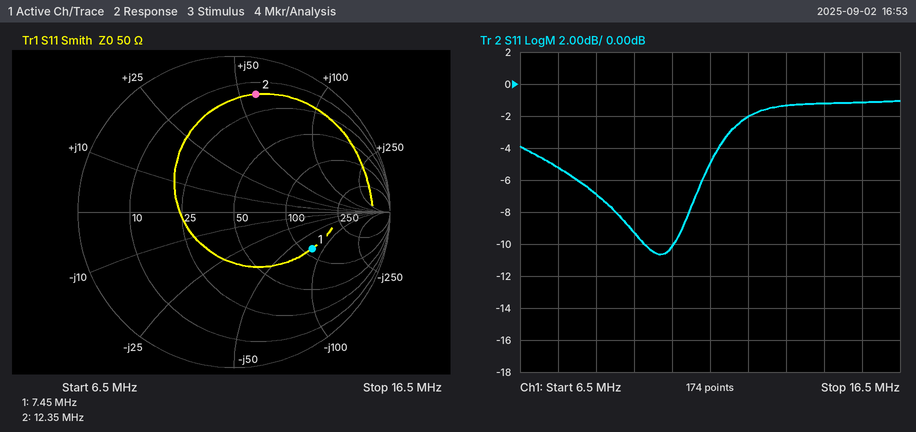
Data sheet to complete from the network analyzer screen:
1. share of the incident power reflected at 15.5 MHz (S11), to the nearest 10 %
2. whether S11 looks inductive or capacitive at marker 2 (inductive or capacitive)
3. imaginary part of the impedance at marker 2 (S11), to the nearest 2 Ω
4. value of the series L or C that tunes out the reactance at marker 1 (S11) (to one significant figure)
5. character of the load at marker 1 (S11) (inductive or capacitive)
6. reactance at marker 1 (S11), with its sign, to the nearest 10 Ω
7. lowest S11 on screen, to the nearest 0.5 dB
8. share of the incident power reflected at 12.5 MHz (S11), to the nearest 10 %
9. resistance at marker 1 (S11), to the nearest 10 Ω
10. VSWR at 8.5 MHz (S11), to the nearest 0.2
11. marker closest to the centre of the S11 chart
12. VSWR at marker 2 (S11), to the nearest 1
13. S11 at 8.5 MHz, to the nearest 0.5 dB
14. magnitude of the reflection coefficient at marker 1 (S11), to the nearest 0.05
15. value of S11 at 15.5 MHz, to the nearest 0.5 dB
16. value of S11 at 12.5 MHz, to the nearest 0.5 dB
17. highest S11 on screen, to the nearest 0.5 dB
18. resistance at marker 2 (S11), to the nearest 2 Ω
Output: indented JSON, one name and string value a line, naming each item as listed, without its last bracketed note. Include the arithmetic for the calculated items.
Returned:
{
  "share of the incident power reflected at 15.5 MHz (S11), to the nearest 10 %": "10^(-1/10) ≈ 79.4 %, so 80 % to the nearest 10 %",
  "whether S11 looks inductive or capacitive at marker 2": "inductive",
  "imaginary part of the impedance at marker 2 (S11), to the nearest 2 Ω": "+58 Ω",
  "value of the series L or C that tunes out the reactance at marker 1 (S11)": "L = 80 Ω/(2π × 7.45 MHz) ≈ 2 µH",
  "character of the load at marker 1 (S11)": "capacitive",
  "reactance at marker 1 (S11), with its sign, to the nearest 10 Ω": "-80 Ω",
  "lowest S11 on screen, to the nearest 0.5 dB": "-10.5 dB",
  "share of the incident power reflected at 12.5 MHz (S11), to the nearest 10 %": "10^(-2/10) ≈ 63.1 %, so 60 % to the nearest 10 %",
  "resistance at marker 1 (S11), to the nearest 10 Ω": "110 Ω",
  "VSWR at 8.5 MHz (S11), to the nearest 0.2": "|Γ| = 10^(-7/20) = 0.4467; VSWR = (1 + 0.4467)/(1 − 0.4467) ≈ 2.6",
  "marker closest to the centre of the S11 chart": "marker 1",
  "VSWR at marker 2 (S11), to the nearest 1": "8",
  "S11 at 8.5 MHz, to the nearest 0.5 dB": "-7.0 dB",
  "magnitude of the reflection coefficient at marker 1 (S11), to the nearest 0.05": "0.55",
  "value of S11 at 15.5 MHz, to the nearest 0.5 dB": "-1.0 dB",
  "value of S11 at 12.5 MHz, to the nearest 0.5 dB": "-2.0 dB",
  "highest S11 on screen, to the nearest 0.5 dB": "-1.0 dB",
  "resistance at marker 2 (S11), to the nearest 2 Ω": "16 Ω"
}
